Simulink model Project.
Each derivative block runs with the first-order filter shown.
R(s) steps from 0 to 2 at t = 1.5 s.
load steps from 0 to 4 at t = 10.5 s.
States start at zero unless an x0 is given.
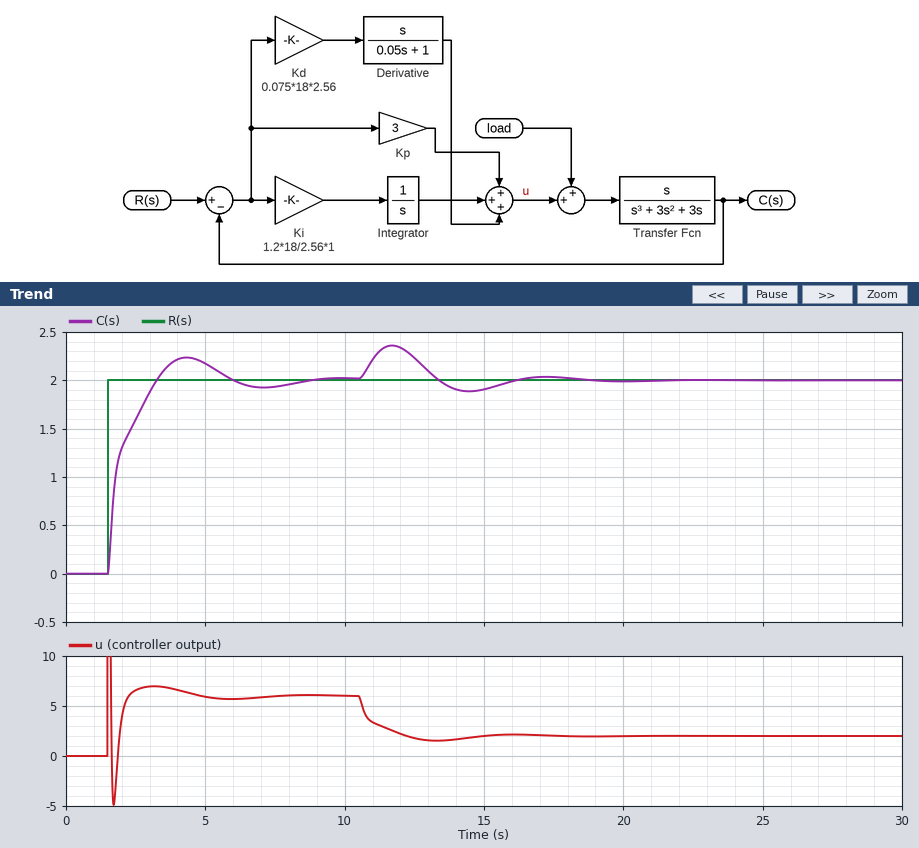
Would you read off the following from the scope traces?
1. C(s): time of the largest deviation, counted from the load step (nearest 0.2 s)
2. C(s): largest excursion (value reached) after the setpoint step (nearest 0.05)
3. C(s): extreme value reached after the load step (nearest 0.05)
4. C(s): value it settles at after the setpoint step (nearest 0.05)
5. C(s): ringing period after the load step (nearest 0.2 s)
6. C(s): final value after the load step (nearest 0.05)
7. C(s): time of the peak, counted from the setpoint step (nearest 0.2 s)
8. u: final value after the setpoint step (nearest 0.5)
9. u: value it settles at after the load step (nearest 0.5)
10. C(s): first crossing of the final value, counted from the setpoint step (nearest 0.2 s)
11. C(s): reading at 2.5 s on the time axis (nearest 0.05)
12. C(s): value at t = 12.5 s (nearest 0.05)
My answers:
1.2 s
2.25
2.35
2.00
5.6 s
2.00
2.8 s
6.0
2.0
1.8 s
1.60
2.25
